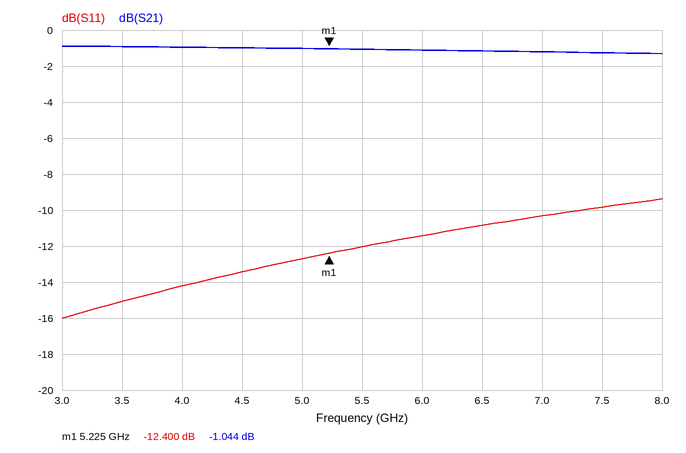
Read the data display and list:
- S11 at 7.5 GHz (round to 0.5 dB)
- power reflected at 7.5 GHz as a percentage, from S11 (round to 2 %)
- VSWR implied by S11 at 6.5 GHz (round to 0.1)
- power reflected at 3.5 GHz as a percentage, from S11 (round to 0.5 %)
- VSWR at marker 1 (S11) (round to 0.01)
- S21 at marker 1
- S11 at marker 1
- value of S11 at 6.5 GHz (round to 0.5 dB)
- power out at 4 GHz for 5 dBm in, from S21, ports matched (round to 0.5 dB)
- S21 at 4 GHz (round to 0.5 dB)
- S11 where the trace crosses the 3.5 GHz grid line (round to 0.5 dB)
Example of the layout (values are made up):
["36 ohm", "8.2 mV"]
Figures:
["-10.0 dB", "10 %", "1.8", "3.0 %", "1.63", "-1.044 dB", "-12.400 dB", "-11.0 dB", "4.0 dBm", "-1.0 dB", "-15.0 dB"]
